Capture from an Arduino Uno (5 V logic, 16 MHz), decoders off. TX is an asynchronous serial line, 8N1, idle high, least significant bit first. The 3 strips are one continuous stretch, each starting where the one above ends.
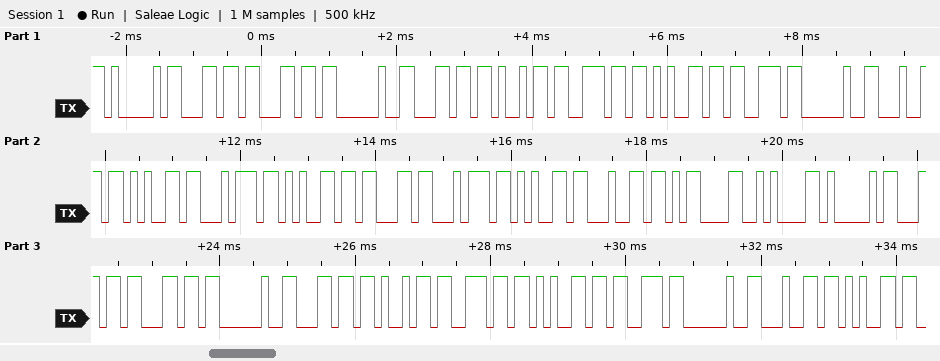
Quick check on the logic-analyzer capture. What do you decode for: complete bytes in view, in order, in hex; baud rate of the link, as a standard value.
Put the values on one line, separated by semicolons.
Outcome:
0x41 0x6C 0x6C 0x20 0x6C 0x69 0x6E 0x65 0x73 0x20 0x64 0x65 0x74 0x65 0x63 0x74 0x65 0x64 0x0D 0x0A 0x41 0x6C 0x6C 0x20 0x6C 0x69 0x6E 0x65 0x73 0x20 0x64 0x65; 9600 baud
